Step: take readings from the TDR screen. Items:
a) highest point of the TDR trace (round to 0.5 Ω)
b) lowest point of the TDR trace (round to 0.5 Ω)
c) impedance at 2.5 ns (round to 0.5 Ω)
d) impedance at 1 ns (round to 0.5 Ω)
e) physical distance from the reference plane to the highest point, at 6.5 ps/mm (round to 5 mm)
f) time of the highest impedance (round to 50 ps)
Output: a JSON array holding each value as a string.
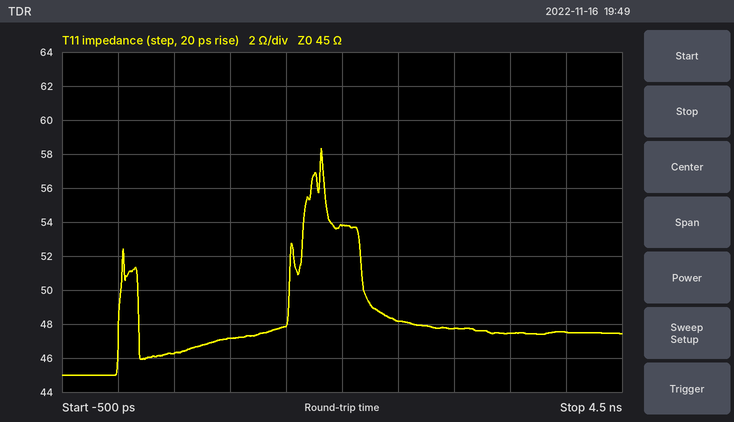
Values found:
["58.5 Ω", "45.0 Ω", "48.0 Ω", "47.0 Ω", "140 mm", "1.80 ns"]
